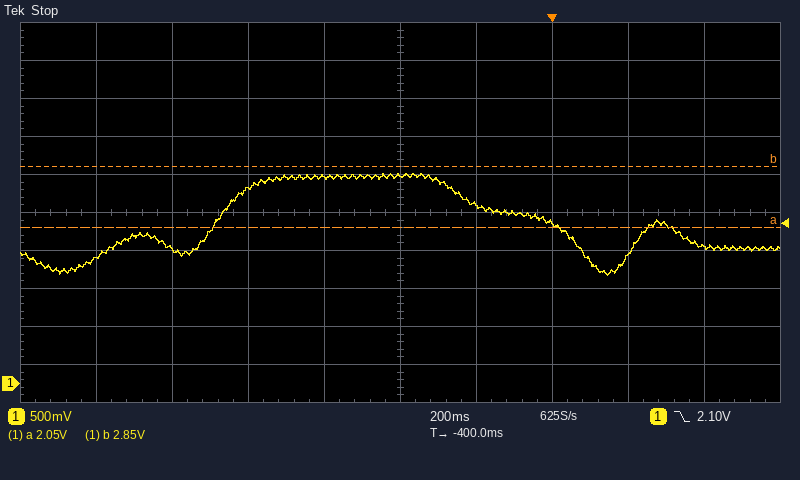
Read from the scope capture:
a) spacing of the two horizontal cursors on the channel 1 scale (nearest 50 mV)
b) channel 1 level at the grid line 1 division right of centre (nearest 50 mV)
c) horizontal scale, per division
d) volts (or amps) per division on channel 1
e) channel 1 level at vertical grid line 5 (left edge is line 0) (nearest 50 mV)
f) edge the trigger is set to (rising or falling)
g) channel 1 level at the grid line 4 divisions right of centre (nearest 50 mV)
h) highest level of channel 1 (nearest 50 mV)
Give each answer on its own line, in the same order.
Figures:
800 mV
2.35 V
200 ms
500 mV
2.75 V
falling
1.80 V
2.75 V
